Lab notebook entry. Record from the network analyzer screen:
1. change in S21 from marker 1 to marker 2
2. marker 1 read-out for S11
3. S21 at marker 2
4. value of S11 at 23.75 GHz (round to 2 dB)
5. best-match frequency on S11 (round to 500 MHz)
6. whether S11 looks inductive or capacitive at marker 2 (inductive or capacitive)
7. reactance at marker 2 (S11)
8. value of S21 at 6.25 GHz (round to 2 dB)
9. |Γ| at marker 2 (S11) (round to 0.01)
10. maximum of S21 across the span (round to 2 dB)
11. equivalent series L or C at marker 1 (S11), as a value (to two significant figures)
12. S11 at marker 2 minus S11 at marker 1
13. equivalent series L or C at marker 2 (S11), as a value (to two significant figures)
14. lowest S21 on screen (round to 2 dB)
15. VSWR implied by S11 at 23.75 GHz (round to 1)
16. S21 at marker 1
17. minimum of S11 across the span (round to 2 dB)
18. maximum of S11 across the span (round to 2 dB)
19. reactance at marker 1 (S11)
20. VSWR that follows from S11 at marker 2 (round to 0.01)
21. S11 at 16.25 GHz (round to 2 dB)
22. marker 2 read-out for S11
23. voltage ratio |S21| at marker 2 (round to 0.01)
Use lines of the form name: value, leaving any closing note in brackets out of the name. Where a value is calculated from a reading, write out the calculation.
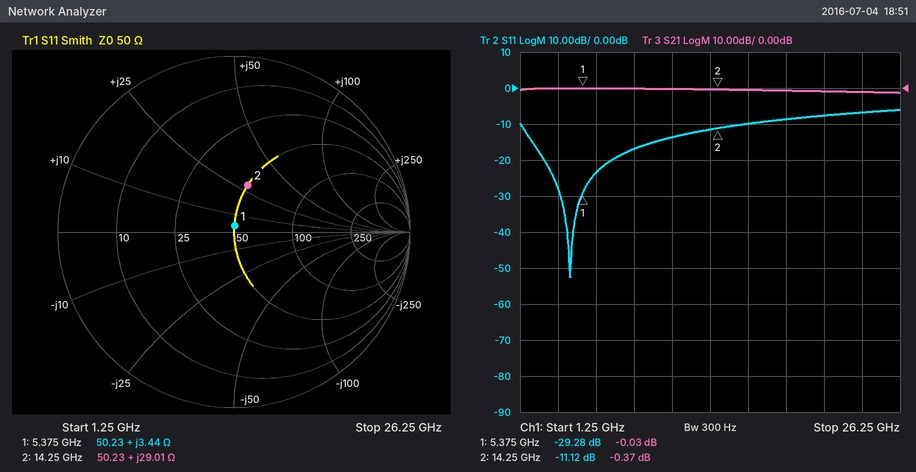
change in S21 from marker 1 to marker 2: -0.37 − (-0.03) = -0.34 dB
marker 1 read-out for S11: -29.28 dB
S21 at marker 2: -0.37 dB
value of S11 at 23.75 GHz: -6 dB
best-match frequency on S11: 4.5 GHz
whether S11 looks inductive or capacitive at marker 2: inductive
reactance at marker 2: +29.01 Ω
value of S21 at 6.25 GHz: 0 dB
|Γ| at marker 2 (S11): 0.28
maximum of S21 across the span: 0 dB
equivalent series L or C at marker 1 (S11), as a value: L = 3.44 Ω/(2π × 5.375 GHz) ≈ 102 pH, so 100 pH to two significant figures
S11 at marker 2 minus S11 at marker 1: -11.12 − (-29.28) = 18.16 dB
equivalent series L or C at marker 2 (S11), as a value: L = 29.01 Ω/(2π × 14.25 GHz) ≈ 324 pH, so 320 pH to two significant figures
lowest S21 on screen: -2 dB
VSWR implied by S11 at 23.75 GHz: |Γ| = 10^(-6/20) = 0.5012; VSWR = (1 + 0.5012)/(1 − 0.5012) ≈ 3
S21 at marker 1: -0.03 dB
minimum of S11 across the span: -52 dB
maximum of S11 across the span: -6 dB
reactance at marker 1: +3.44 Ω
VSWR that follows from S11 at marker 2: (1 + 0.2780)/(1 − 0.2780) ≈ 1.77
S11 at 16.25 GHz: -10 dB
marker 2 read-out for S11: -11.12 dB
voltage ratio |S21| at marker 2: 10^(-0.37/20) ≈ 0.96
